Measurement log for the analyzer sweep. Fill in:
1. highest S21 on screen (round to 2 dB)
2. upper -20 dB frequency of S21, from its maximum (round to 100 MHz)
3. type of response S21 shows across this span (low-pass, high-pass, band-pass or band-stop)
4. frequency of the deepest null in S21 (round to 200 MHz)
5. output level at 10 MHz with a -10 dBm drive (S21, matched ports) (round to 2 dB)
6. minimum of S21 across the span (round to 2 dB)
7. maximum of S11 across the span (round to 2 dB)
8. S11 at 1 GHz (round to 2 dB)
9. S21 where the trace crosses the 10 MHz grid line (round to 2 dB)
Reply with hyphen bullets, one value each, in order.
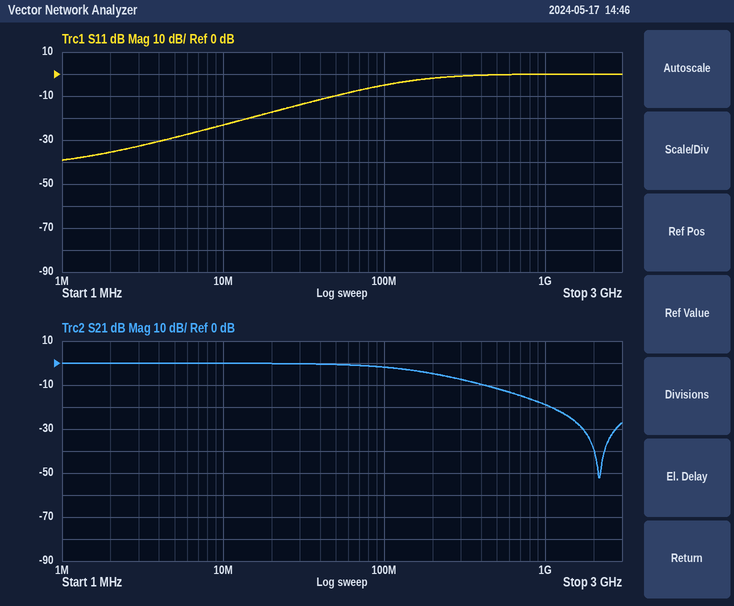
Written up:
- 0 dB
- 1.1 GHz
- low-pass
- 2.2 GHz
- -10 dBm
- -52 dB
- 0 dB
- 0 dB
- 0 dB
